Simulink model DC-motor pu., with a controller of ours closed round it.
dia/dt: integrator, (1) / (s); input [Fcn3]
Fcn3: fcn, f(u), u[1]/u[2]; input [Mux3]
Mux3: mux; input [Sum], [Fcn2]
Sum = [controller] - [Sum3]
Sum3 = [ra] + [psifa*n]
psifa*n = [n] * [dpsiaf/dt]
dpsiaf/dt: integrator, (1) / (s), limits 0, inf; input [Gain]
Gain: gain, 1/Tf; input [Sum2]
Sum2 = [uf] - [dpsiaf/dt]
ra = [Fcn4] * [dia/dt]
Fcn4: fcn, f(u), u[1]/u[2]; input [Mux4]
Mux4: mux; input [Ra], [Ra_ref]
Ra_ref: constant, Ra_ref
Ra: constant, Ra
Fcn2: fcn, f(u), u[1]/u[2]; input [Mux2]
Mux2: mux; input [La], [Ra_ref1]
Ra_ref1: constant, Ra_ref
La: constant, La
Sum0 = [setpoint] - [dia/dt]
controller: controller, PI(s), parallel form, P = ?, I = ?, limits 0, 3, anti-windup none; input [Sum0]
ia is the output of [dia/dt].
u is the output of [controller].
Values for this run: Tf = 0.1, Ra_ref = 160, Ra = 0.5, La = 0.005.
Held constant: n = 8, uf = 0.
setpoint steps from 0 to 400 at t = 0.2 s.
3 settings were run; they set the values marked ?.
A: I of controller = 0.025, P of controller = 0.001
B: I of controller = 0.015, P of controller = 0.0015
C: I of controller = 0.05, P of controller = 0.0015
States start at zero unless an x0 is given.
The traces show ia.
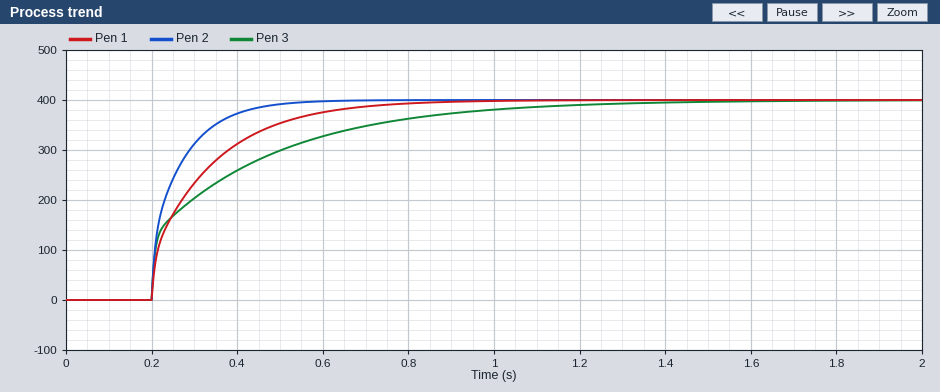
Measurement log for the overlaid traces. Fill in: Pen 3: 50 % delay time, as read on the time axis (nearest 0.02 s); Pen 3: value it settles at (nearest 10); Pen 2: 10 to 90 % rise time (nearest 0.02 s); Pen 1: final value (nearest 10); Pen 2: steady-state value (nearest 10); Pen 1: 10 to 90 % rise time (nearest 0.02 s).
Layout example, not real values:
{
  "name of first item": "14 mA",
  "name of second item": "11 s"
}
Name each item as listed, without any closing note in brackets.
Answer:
{
  "Pen 3: 50 % delay time, as read on the time axis": "0.30 s",
  "Pen 3: value it settles at": "400",
  "Pen 2: 10 to 90 % rise time": "0.16 s",
  "Pen 1: final value": "400",
  "Pen 2: steady-state value": "400",
  "Pen 1: 10 to 90 % rise time": "0.32 s"
}
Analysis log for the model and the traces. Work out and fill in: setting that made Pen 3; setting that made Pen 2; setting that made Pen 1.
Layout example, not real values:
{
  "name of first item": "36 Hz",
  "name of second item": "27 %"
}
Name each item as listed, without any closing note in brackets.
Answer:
{
  "setting that made Pen 3": "B",
  "setting that made Pen 2": "C",
  "setting that made Pen 1": "A"
}
